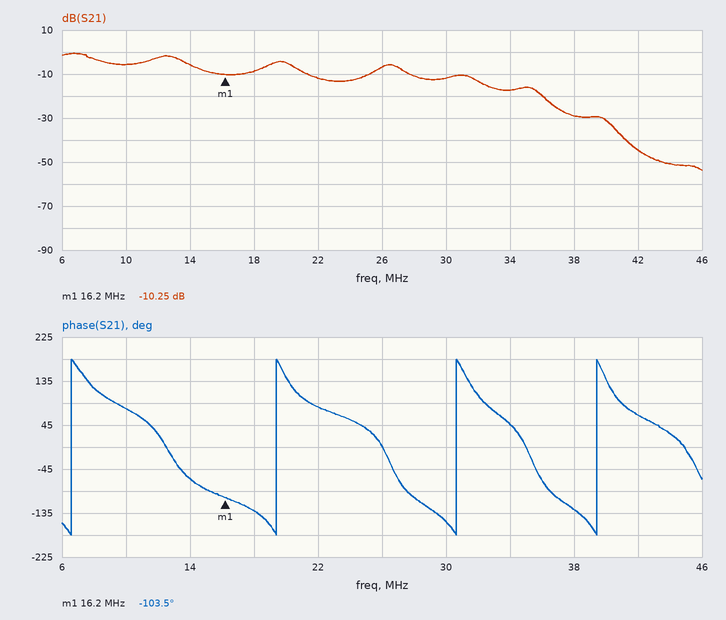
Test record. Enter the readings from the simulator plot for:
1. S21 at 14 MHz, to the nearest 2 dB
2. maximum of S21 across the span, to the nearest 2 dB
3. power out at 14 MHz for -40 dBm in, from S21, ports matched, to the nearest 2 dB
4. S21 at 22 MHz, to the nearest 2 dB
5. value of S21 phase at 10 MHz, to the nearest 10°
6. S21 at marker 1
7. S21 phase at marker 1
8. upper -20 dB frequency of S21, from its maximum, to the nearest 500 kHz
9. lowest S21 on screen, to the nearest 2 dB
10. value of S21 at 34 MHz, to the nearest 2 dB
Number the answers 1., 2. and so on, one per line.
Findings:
1. -6 dB
2. 0 dB
3. -46 dBm
4. -12 dB
5. 80°
6. -10.25 dB
7. -103.5°
8. 36.0 MHz
9. -54 dB
10. -18 dB
